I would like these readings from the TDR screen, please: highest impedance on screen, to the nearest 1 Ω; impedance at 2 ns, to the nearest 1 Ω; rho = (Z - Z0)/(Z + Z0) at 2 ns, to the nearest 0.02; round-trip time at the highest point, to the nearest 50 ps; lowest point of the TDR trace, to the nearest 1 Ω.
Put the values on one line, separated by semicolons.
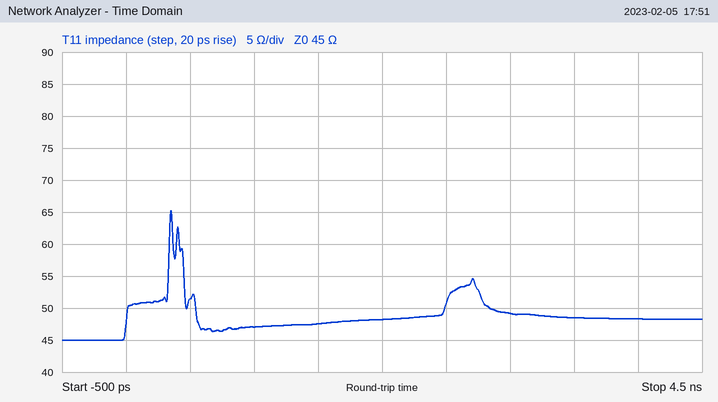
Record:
65 Ω; 48 Ω; +0.04; 350 ps; 45 Ω
